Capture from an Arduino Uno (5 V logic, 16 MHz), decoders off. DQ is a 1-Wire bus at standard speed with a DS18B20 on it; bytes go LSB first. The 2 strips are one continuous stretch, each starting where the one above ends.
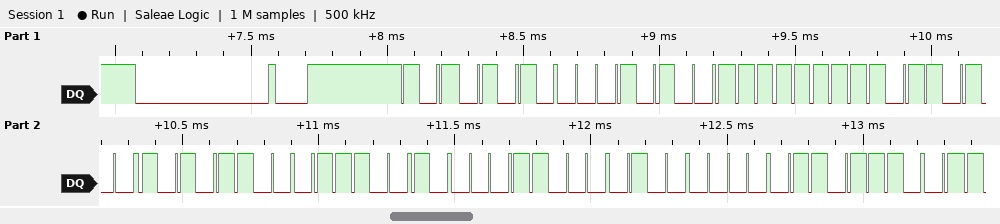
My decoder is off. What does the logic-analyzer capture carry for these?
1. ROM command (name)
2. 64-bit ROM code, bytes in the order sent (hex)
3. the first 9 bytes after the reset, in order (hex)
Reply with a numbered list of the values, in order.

1. Match ROM
2. 28 FF 2D 35 4E 18 02 76
3. 55 28 FF 2D 35 4E 18 02 76
